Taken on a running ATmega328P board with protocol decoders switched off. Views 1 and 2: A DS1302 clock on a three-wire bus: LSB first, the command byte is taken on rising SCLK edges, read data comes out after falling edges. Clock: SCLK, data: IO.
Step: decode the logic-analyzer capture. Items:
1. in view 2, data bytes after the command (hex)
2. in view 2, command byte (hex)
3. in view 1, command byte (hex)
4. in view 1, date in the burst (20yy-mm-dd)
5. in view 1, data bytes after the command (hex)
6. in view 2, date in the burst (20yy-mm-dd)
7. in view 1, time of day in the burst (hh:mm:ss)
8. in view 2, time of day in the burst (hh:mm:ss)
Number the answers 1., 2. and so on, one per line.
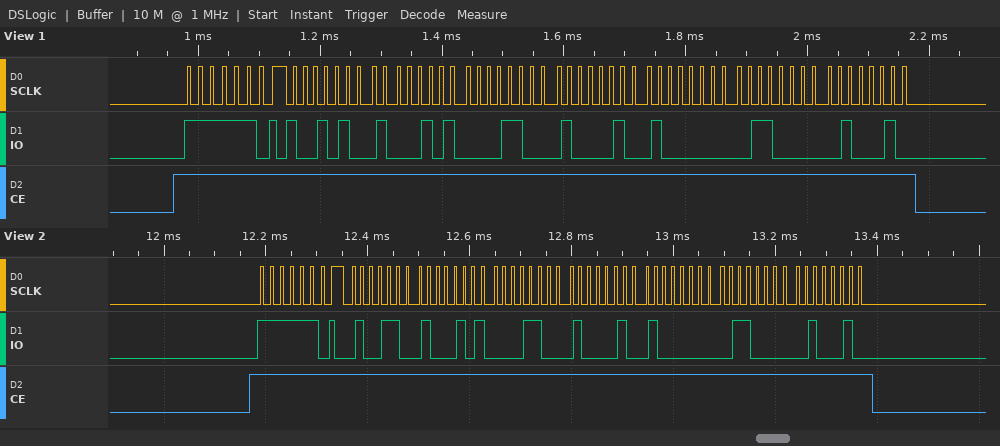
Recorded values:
1. 32 51 18 21 01 06 22
2. 0xBF
3. 0xBF
4. 2022-01-21
5. 29 51 18 21 01 06 22
6. 2022-01-21
7. 18:51:29
8. 18:51:32
